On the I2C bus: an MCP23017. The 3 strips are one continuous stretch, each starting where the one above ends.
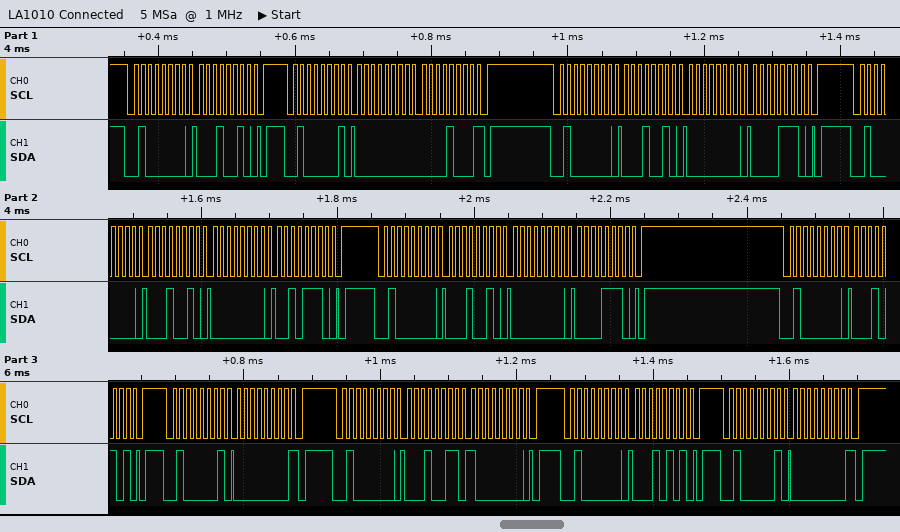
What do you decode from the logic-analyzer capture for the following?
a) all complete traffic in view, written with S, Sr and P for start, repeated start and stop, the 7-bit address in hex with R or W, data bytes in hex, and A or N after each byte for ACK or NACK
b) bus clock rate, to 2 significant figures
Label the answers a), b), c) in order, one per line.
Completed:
a) S 20W A 12 A P S 20R A 00 A 08 N P S 20W A 12 A 00 A 0E A P S 20W A 12 A 00 A 2E A P S 20W A 12 A 00 A 0E A P S 20W A 15 A P S 20R A 00 N P S 20W A 13 A 80 A P S 20W A 15 A P S 20R A 00 N P
b) 100 kHz
